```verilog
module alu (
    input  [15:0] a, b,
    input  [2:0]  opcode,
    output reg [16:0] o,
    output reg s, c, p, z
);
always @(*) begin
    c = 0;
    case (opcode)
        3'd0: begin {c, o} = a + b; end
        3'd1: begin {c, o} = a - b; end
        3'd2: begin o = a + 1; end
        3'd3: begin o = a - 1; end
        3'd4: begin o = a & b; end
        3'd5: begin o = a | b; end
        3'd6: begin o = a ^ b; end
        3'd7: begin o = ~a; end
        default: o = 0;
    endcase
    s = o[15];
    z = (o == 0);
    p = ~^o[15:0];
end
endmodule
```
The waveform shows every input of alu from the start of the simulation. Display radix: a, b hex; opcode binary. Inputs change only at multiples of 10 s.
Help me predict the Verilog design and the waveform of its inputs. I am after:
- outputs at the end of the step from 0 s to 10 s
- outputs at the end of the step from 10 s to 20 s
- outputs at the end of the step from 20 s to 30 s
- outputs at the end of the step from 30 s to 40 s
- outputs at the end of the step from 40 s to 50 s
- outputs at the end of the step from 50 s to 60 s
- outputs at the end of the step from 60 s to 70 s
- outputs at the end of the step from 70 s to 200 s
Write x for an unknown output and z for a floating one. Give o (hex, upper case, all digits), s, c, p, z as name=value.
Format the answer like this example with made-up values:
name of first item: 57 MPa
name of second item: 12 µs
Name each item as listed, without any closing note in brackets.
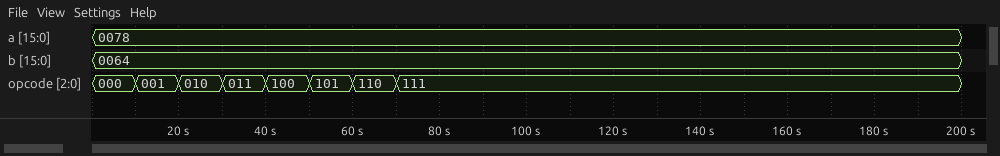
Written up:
outputs at the end of the step from 0 s to 10 s: o=000DC, s=0, c=0, p=0, z=0
outputs at the end of the step from 10 s to 20 s: o=00014, s=0, c=0, p=1, z=0
outputs at the end of the step from 20 s to 30 s: o=00079, s=0, c=0, p=0, z=0
outputs at the end of the step from 30 s to 40 s: o=00077, s=0, c=0, p=1, z=0
outputs at the end of the step from 40 s to 50 s: o=00060, s=0, c=0, p=1, z=0
outputs at the end of the step from 50 s to 60 s: o=0007C, s=0, c=0, p=0, z=0
outputs at the end of the step from 60 s to 70 s: o=0001C, s=0, c=0, p=0, z=0
outputs at the end of the step from 70 s to 200 s: o=1FF87, s=1, c=0, p=1, z=0
